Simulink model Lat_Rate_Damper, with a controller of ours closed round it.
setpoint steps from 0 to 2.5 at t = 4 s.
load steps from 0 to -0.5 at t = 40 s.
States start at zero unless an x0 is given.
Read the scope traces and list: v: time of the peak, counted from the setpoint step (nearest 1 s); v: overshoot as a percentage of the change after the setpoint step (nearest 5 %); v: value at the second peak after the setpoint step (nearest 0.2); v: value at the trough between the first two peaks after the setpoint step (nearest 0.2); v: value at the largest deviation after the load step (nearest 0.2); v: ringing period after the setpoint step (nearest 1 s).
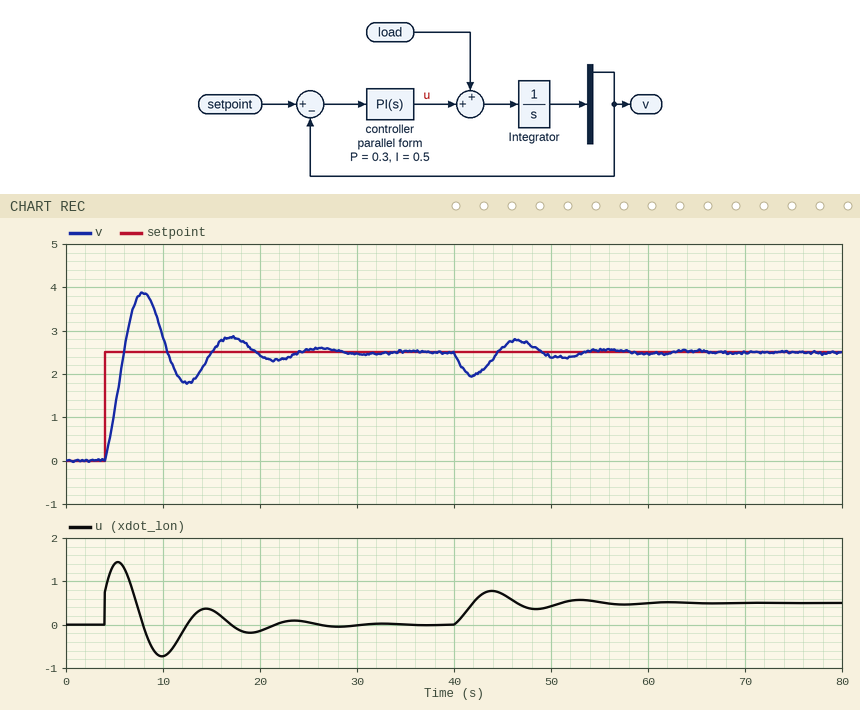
4 s
55 %
2.8
1.8
2.0
9 s
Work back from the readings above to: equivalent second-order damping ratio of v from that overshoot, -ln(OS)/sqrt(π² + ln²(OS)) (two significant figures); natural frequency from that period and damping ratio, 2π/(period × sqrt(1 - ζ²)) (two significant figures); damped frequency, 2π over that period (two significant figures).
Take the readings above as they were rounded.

0.19
0.71 rad/s
0.70 rad/s
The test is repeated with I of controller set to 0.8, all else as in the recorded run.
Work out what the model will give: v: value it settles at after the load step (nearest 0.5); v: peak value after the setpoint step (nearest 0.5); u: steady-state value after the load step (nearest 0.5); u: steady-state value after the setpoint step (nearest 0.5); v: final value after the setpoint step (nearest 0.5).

2.5
4.0
0.5
0.0
2.5
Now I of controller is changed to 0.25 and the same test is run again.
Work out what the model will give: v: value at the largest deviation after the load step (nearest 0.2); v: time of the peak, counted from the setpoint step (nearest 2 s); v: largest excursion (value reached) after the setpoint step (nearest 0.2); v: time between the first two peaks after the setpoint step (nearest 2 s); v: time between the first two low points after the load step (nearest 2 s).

1.8
6 s
3.6
14 s
14 s
